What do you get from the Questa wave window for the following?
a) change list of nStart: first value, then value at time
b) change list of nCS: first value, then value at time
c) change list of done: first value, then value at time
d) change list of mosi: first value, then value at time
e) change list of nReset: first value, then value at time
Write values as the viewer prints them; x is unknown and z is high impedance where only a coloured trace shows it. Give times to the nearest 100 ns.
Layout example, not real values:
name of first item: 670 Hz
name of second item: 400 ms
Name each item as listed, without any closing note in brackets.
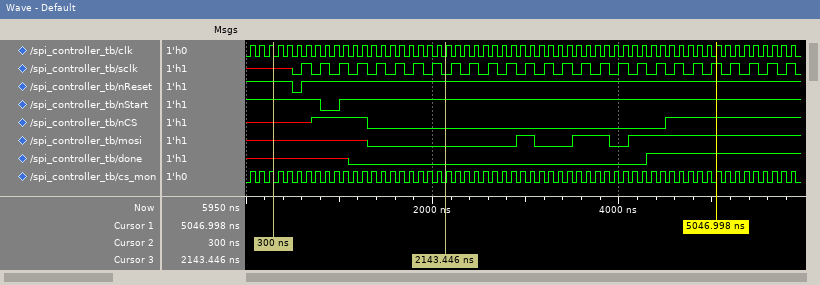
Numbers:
change list of nStart: first value, then value at time: 1, 0 at 800 ns, 1 at 1000 ns
change list of nCS: first value, then value at time: x, 1 at 700 ns, 0 at 1300 ns, 1 at 4500 ns
change list of done: first value, then value at time: x, 0 at 1100 ns, 1 at 4300 ns
change list of mosi: first value, then value at time: x, 0 at 1300 ns, 1 at 2900 ns, 0 at 3100 ns, 1 at 3500 ns, 0 at 3900 ns, 1 at 4100 ns
change list of nReset: first value, then value at time: 1, 0 at 500 ns, 1 at 600 ns
